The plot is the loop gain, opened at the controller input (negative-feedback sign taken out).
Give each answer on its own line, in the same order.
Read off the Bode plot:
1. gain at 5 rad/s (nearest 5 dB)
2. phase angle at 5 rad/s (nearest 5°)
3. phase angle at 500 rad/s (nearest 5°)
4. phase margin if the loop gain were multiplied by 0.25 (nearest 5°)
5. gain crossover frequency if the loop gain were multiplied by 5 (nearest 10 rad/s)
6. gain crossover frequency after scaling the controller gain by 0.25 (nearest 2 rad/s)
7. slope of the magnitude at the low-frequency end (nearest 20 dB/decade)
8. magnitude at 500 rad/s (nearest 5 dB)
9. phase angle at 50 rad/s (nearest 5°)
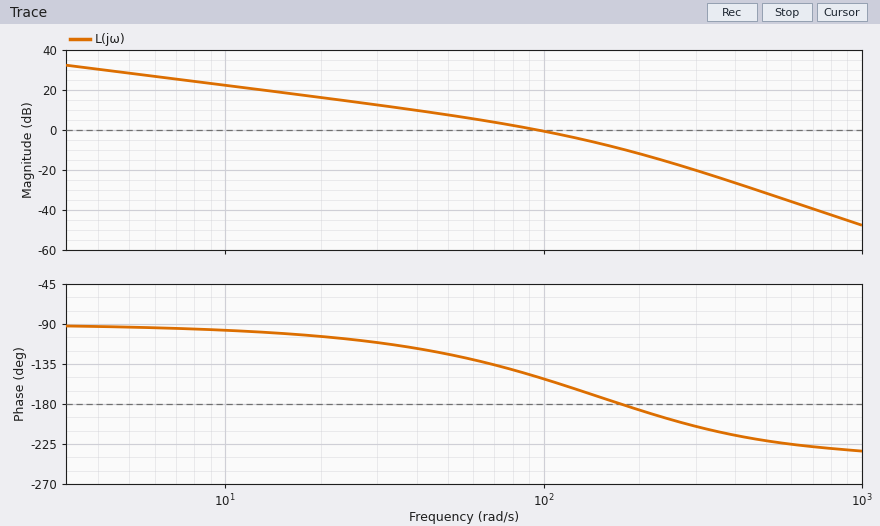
30 dB
-95°
-220°
70°
220 rad/s
32 rad/s
-20 dB/decade
-30 dB
-125°
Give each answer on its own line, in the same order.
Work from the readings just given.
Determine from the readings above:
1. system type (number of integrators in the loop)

1
